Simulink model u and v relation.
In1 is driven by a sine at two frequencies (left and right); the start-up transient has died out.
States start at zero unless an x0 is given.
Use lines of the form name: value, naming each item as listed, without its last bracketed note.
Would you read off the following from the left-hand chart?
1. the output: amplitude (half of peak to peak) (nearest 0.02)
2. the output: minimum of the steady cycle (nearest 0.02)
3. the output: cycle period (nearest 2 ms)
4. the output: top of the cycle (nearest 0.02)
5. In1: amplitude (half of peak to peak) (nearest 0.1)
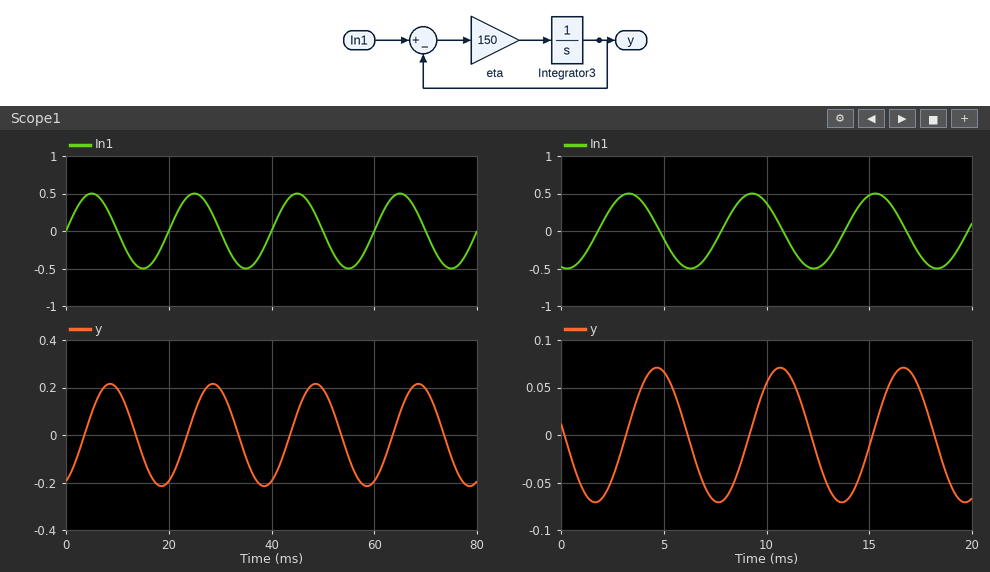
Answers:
the output: amplitude (half of peak to peak): 0.22
the output: minimum of the steady cycle: -0.22
the output: cycle period: 20 ms
the output: top of the cycle: 0.22
In1: amplitude (half of peak to peak): 0.5
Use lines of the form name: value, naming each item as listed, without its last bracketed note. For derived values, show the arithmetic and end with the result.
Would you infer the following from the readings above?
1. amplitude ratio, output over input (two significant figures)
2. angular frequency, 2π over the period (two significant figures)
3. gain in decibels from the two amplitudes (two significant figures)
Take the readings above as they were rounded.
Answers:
amplitude ratio, output over input: 0.22 / 0.5 = 0.44
angular frequency, 2π over the period: 2π / 20 = 0.31 rad/ms
gain in decibels from the two amplitudes: 20 log10(0.22 / 0.5) = -7.1 dB
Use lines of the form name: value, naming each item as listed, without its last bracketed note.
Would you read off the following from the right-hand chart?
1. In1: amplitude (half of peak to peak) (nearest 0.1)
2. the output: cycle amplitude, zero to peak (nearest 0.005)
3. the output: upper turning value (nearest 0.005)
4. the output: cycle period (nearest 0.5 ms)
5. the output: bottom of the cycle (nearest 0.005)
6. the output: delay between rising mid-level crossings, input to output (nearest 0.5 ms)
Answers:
In1: amplitude (half of peak to peak): 0.5
the output: cycle amplitude, zero to peak: 0.070
the output: upper turning value: 0.070
the output: cycle period: 6.0 ms
the output: bottom of the cycle: -0.070
the output: delay between rising mid-level crossings, input to output: 1.5 ms
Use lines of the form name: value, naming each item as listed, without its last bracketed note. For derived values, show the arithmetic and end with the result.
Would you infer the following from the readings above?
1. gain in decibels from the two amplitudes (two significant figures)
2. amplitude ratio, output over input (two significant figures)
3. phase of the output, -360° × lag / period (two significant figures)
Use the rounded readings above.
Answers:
gain in decibels from the two amplitudes: 20 log10(0.07 / 0.5) = -17 dB
amplitude ratio, output over input: 0.07 / 0.5 = 0.14
phase of the output, -360° × lag / period: -360 × 1.5 / 6 = -90°
